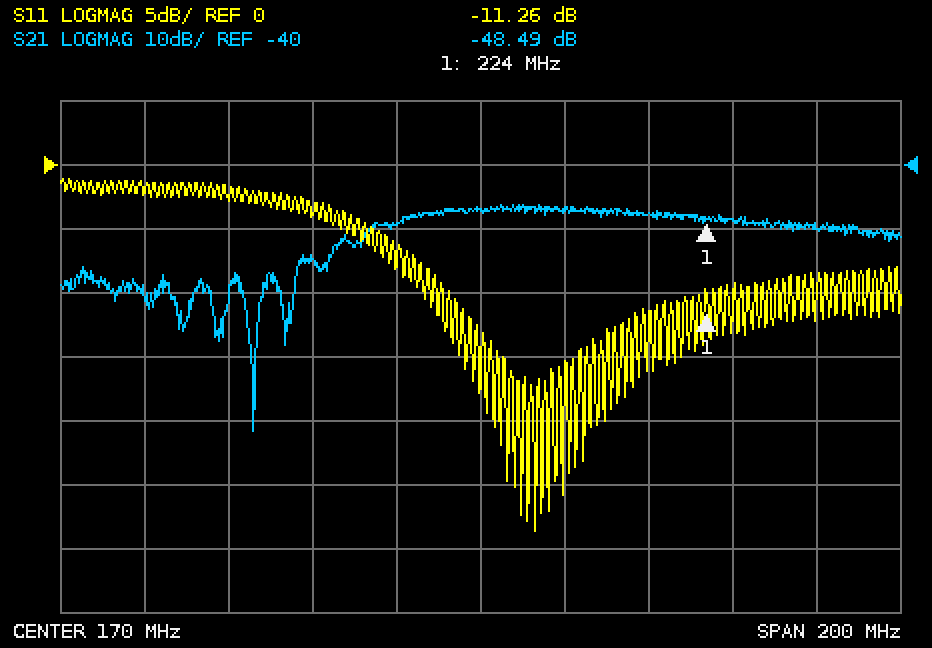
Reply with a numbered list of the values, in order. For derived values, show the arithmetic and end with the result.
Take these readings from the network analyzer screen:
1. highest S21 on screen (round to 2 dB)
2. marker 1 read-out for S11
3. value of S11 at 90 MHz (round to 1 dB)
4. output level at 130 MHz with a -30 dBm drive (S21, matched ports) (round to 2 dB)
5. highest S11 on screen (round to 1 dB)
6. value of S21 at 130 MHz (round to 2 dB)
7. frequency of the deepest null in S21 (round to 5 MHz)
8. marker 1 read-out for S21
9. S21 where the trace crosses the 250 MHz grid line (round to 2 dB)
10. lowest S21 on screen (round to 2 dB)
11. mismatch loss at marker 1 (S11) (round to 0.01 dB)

1. -46 dB
2. -11.26 dB
3. -2 dB
4. -30 dBm + (-54 dB) = -84 dBm
5. -1 dB
6. -54 dB
7. 115 MHz
8. -48.49 dB
9. -50 dB
10. -82 dB
11. −10 log10(1 − 10^(-11.26/10)) ≈ 0.34 dB
